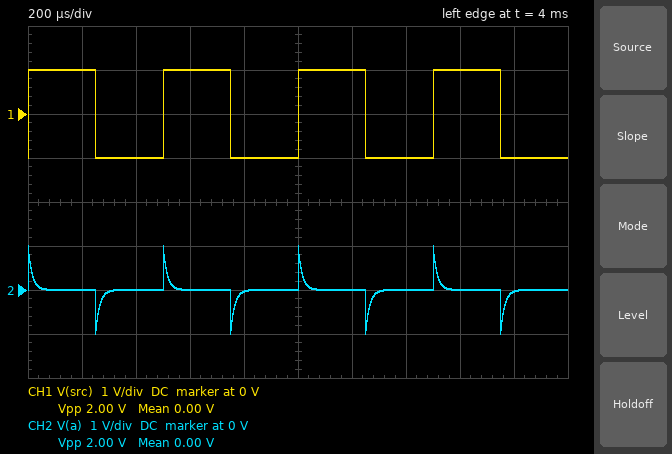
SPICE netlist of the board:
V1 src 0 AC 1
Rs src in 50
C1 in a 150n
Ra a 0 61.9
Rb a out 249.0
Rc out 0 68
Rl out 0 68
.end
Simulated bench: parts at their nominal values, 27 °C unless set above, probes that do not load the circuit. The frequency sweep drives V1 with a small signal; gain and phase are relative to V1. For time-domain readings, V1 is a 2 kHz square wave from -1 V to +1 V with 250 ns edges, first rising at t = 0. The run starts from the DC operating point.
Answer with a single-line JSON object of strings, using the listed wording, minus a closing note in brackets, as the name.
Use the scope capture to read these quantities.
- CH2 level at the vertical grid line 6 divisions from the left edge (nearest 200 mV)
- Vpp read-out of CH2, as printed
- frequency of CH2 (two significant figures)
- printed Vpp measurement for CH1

{"CH2 level at the vertical grid line 6 divisions from the left edge": "0 V", "Vpp read-out of CH2, as printed": "2.00 V", "frequency of CH2": "2.0 kHz", "printed Vpp measurement for CH1": "2.00 V"}
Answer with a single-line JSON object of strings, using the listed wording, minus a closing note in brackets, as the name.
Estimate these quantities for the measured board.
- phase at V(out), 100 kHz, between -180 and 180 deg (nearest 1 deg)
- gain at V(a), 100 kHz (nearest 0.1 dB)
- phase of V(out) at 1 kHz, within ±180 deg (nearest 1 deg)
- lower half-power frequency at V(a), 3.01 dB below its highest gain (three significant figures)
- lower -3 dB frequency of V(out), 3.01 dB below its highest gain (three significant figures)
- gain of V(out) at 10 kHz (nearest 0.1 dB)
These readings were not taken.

{"phase at V(out), 100 kHz, between -180 and 180 deg": "6 deg", "gain at V(a), 100 kHz": "-6.0 dB", "phase of V(out) at 1 kHz, within ±180 deg": "85 deg", "lower half-power frequency at V(a), 3.01 dB below its highest gain": "10.5 kHz", "lower -3 dB frequency of V(out), 3.01 dB below its highest gain": "10.5 kHz", "gain of V(out) at 10 kHz": "-27.6 dB"}
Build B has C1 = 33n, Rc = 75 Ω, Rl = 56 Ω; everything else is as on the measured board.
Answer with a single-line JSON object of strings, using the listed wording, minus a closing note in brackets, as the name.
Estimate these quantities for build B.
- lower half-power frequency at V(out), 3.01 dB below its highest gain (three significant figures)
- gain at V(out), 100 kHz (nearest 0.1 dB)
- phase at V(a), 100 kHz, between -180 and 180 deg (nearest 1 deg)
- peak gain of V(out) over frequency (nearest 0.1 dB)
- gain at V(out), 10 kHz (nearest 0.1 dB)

{"lower half-power frequency at V(out), 3.01 dB below its highest gain": "47.9 kHz", "gain at V(out), 100 kHz": "-25.7 dB", "phase at V(a), 100 kHz, between -180 and 180 deg": "26 deg", "peak gain of V(out) over frequency": "-24.8 dB", "gain at V(out), 10 kHz": "-38.6 dB"}
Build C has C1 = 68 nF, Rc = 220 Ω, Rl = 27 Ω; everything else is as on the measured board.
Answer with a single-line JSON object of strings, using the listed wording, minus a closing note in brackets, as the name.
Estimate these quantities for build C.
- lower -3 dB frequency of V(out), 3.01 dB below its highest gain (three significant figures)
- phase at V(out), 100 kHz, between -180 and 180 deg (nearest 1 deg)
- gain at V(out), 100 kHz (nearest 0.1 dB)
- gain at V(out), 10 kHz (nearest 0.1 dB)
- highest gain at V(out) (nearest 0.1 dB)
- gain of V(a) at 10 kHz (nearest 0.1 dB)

{"lower -3 dB frequency of V(out), 3.01 dB below its highest gain": "23.3 kHz", "phase at V(out), 100 kHz, between -180 and 180 deg": "13 deg", "gain at V(out), 100 kHz": "-27.3 dB", "gain at V(out), 10 kHz": "-35.2 dB", "highest gain at V(out)": "-27.1 dB", "gain of V(a) at 10 kHz": "-14.1 dB"}
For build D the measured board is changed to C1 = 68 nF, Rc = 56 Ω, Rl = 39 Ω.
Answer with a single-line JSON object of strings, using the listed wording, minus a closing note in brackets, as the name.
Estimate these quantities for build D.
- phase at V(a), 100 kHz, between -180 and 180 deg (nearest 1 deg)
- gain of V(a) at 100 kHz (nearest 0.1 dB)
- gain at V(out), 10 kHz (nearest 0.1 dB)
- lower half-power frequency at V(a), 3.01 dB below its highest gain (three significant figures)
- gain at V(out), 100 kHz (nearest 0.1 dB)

{"phase at V(a), 100 kHz, between -180 and 180 deg": "13 deg", "gain of V(a) at 100 kHz": "-6.2 dB", "gain at V(out), 10 kHz": "-35.5 dB", "lower half-power frequency at V(a), 3.01 dB below its highest gain": "23.3 kHz", "gain at V(out), 100 kHz": "-27.7 dB"}
